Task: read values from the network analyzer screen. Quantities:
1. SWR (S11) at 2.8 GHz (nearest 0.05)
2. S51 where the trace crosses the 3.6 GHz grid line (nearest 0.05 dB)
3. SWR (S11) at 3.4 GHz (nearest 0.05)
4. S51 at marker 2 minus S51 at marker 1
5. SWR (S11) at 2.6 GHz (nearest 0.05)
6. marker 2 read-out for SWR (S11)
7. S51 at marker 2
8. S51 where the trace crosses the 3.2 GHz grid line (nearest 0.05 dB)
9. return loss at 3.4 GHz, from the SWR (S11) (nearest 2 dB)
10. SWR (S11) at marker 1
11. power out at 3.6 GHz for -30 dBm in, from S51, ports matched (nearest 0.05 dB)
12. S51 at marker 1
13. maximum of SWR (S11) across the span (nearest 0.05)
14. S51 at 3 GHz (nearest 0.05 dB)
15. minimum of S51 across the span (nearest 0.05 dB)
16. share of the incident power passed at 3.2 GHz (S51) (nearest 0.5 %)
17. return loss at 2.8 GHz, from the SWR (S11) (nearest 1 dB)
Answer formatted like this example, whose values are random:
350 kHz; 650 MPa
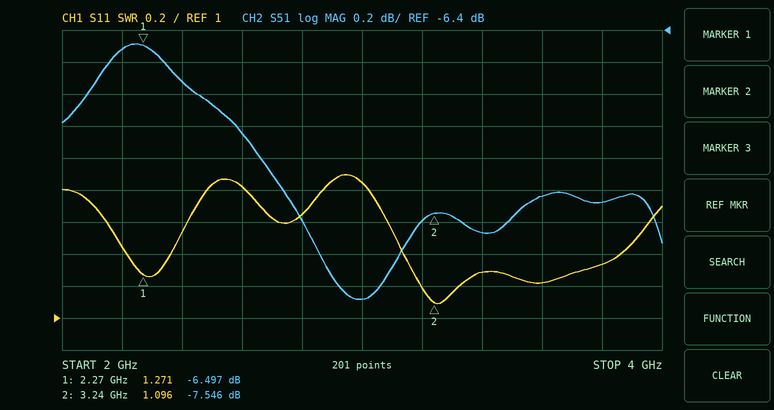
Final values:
1.65; -7.45 dB; 1.30; -1.049 dB; 1.80; 1.096; -7.546 dB; -7.60 dB; 18 dB; 1.271; -37.45 dBm; -6.497 dB; 1.90; -8.10 dB; -8.10 dB; 17.5 %; 12 dB
